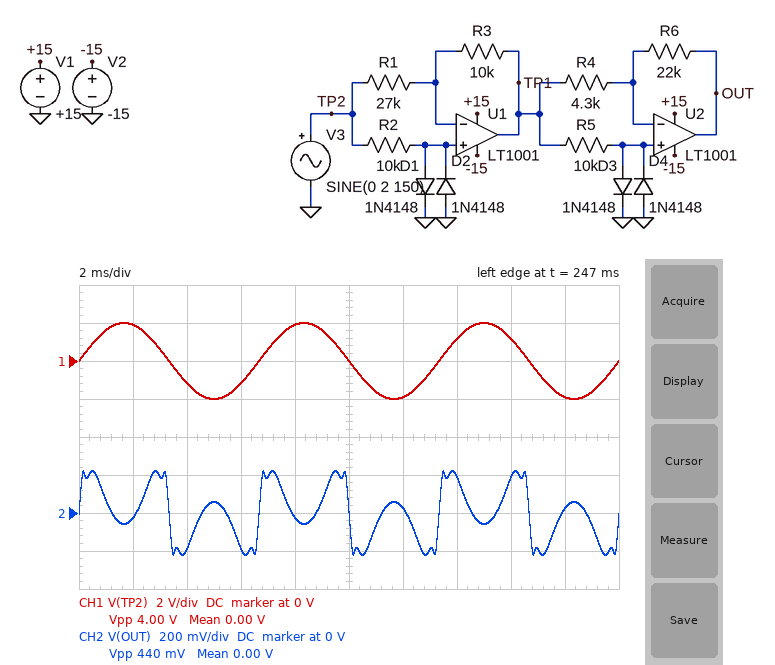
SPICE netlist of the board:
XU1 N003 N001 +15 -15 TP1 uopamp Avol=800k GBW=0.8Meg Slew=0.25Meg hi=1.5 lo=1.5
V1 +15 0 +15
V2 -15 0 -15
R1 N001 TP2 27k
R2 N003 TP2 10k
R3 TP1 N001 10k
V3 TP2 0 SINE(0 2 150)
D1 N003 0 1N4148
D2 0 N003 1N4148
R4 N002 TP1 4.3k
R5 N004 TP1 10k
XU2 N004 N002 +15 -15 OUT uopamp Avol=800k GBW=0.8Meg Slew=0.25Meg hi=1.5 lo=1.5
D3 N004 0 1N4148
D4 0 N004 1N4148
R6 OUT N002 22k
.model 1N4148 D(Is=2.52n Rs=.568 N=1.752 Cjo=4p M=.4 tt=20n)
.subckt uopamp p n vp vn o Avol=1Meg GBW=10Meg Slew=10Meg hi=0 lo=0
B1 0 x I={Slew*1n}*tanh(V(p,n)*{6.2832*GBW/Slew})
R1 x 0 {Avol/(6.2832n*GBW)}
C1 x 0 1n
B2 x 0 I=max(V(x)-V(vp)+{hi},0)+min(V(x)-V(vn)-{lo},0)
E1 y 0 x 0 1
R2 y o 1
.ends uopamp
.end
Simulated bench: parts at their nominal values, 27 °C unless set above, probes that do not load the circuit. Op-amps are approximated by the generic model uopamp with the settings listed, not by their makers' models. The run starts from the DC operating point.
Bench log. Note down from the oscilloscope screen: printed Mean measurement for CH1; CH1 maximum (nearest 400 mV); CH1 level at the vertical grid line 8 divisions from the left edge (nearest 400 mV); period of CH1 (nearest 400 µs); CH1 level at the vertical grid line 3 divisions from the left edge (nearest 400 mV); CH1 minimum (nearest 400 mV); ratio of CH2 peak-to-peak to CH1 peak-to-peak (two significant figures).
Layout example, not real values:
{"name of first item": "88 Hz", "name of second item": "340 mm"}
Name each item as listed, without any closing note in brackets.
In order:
{"printed Mean measurement for CH1": "0.00 V", "CH1 maximum": "2.0 V", "CH1 level at the vertical grid line 8 divisions from the left edge": "1.2 V", "period of CH1": "6.8 ms", "CH1 level at the vertical grid line 3 divisions from the left edge": "-1.2 V", "CH1 minimum": "-2.0 V", "ratio of CH2 peak-to-peak to CH1 peak-to-peak": "0.11"}
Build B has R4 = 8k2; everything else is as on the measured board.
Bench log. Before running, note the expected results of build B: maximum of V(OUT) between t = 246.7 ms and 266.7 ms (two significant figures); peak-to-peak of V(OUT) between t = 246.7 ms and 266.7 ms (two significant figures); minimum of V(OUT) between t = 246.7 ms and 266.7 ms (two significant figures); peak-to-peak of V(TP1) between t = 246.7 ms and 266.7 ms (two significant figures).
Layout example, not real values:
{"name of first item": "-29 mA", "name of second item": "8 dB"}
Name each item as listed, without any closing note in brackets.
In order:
{"maximum of V(OUT) between t = 246.7 ms and 266.7 ms": "250 mV", "peak-to-peak of V(OUT) between t = 246.7 ms and 266.7 ms": "500 mV", "minimum of V(OUT) between t = 246.7 ms and 266.7 ms": "-250 mV", "peak-to-peak of V(TP1) between t = 246.7 ms and 266.7 ms": "680 mV"}
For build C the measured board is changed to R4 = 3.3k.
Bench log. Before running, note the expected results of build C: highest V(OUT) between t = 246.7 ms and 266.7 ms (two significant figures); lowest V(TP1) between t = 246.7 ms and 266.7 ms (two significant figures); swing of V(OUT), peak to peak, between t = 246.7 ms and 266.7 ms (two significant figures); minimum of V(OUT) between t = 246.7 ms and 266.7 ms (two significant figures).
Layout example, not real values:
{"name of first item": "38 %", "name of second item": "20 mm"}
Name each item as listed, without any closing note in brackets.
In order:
{"highest V(OUT) between t = 246.7 ms and 266.7 ms": "210 mV", "lowest V(TP1) between t = 246.7 ms and 266.7 ms": "-340 mV", "swing of V(OUT), peak to peak, between t = 246.7 ms and 266.7 ms": "420 mV", "minimum of V(OUT) between t = 246.7 ms and 266.7 ms": "-210 mV"}
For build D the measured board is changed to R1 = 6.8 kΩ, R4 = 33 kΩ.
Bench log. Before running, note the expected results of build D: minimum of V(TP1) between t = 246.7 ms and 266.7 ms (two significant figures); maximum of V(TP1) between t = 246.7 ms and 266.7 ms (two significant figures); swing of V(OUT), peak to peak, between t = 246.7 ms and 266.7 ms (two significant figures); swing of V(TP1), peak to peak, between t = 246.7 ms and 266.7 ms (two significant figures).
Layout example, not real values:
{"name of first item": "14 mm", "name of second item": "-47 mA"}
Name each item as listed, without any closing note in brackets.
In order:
{"minimum of V(TP1) between t = 246.7 ms and 266.7 ms": "-1.7 V", "maximum of V(TP1) between t = 246.7 ms and 266.7 ms": "1.7 V", "swing of V(OUT), peak to peak, between t = 246.7 ms and 266.7 ms": "650 mV", "swing of V(TP1), peak to peak, between t = 246.7 ms and 266.7 ms": "3.4 V"}
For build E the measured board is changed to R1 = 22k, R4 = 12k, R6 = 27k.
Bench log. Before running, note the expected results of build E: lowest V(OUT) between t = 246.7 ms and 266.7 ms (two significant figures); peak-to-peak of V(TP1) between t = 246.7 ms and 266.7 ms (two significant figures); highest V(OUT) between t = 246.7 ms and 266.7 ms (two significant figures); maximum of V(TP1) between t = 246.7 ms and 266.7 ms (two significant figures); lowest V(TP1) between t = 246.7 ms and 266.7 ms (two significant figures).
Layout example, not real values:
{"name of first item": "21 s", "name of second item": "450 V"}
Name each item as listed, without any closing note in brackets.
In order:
{"lowest V(OUT) between t = 246.7 ms and 266.7 ms": "-260 mV", "peak-to-peak of V(TP1) between t = 246.7 ms and 266.7 ms": "660 mV", "highest V(OUT) between t = 246.7 ms and 266.7 ms": "260 mV", "maximum of V(TP1) between t = 246.7 ms and 266.7 ms": "330 mV", "lowest V(TP1) between t = 246.7 ms and 266.7 ms": "-330 mV"}
